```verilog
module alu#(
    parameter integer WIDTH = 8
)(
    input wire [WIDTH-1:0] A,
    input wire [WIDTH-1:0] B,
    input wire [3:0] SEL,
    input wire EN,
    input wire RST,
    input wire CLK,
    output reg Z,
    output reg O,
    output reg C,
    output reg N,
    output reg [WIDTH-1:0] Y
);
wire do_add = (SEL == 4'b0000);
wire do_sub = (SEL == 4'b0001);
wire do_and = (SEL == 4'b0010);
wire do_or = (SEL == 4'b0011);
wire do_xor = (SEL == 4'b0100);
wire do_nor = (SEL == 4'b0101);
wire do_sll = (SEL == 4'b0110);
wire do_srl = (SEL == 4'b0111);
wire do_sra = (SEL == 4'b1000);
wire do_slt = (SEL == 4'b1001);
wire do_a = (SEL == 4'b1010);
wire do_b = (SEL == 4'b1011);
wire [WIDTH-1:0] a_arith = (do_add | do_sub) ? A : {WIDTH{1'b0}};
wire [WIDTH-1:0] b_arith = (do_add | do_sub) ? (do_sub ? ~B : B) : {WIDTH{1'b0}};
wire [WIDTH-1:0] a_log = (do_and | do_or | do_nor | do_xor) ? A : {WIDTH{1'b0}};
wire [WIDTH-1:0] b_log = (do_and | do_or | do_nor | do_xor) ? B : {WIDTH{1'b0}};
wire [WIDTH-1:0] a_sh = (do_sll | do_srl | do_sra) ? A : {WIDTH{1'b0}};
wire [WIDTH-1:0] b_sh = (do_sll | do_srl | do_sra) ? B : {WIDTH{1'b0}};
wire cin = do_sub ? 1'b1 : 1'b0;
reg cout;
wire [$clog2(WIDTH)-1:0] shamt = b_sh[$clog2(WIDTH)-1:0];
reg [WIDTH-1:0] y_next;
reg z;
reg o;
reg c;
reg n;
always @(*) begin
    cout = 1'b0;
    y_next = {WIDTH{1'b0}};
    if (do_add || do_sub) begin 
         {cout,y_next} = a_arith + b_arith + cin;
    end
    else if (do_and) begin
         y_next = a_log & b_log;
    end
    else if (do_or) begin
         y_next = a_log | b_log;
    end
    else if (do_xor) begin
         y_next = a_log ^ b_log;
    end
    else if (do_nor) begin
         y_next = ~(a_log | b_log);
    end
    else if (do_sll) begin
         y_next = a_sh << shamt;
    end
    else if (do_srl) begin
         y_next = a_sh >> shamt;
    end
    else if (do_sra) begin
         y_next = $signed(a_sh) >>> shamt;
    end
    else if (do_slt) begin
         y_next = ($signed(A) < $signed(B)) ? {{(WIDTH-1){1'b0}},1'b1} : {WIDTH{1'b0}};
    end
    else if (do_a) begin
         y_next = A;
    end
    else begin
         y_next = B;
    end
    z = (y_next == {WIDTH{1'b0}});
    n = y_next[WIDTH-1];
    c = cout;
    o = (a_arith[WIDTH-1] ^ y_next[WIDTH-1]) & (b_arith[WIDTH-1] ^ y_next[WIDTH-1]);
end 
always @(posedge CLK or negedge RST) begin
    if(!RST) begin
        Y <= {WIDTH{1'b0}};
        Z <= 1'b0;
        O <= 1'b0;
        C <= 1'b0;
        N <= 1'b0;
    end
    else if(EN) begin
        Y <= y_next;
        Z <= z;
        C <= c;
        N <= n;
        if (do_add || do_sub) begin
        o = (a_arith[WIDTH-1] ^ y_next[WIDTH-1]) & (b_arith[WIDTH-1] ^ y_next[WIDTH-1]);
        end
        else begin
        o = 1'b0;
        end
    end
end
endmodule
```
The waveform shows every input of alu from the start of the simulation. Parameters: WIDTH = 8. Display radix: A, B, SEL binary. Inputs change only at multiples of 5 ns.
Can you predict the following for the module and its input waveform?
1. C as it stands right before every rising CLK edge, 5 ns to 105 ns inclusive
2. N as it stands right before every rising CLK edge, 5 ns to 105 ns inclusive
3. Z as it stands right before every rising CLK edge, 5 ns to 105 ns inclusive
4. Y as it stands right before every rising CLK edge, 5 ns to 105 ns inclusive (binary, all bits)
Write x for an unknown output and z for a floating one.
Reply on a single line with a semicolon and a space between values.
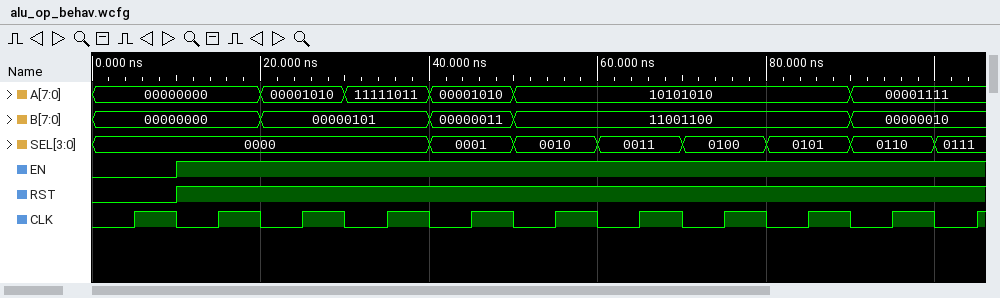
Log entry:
0 0 0 0 1 1 0 0 0 0 0; 0 0 0 0 0 0 1 1 0 0 0; 0 0 1 0 1 0 0 0 0 0 0; 00000000, 00000000, 00000000, 00001111, 00000000, 00000111, 10001000, 11101110, 01100110, 00010001, 00111100
